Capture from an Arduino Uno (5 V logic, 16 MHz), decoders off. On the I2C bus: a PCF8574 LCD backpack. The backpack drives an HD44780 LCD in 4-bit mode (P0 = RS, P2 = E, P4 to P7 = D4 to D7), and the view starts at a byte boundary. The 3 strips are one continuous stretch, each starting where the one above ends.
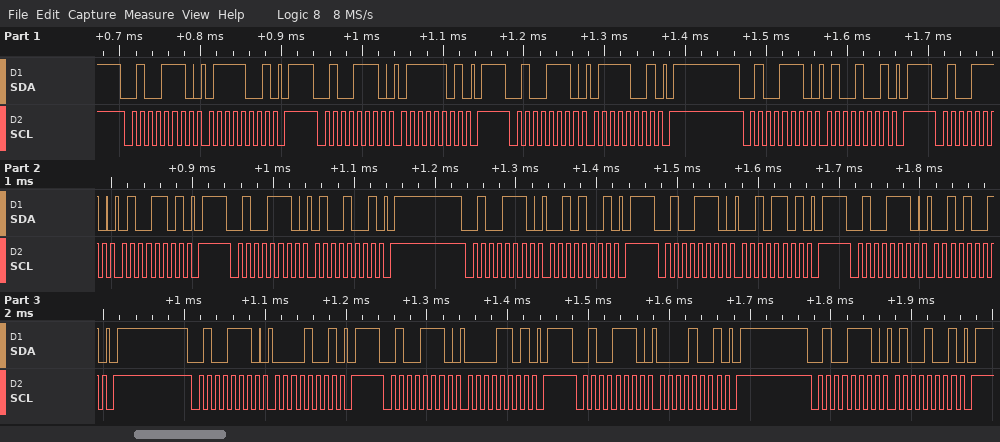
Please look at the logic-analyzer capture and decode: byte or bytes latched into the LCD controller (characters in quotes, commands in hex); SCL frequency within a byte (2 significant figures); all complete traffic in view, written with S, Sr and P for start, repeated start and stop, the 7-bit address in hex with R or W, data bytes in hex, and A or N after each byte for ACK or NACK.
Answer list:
't' ' '
100 kHz
S 27W A 79 A P S 27W A 7D A P S 27W A 79 A P S 27W A 49 A P S 27W A 4D A P S 27W A 49 A P S 27W A 29 A P S 27W A 2D A P S 27W A 29 A P S 27W A 09 A P S 27W A 0D A P S 27W A 09 A P S 27W A 49 A P
